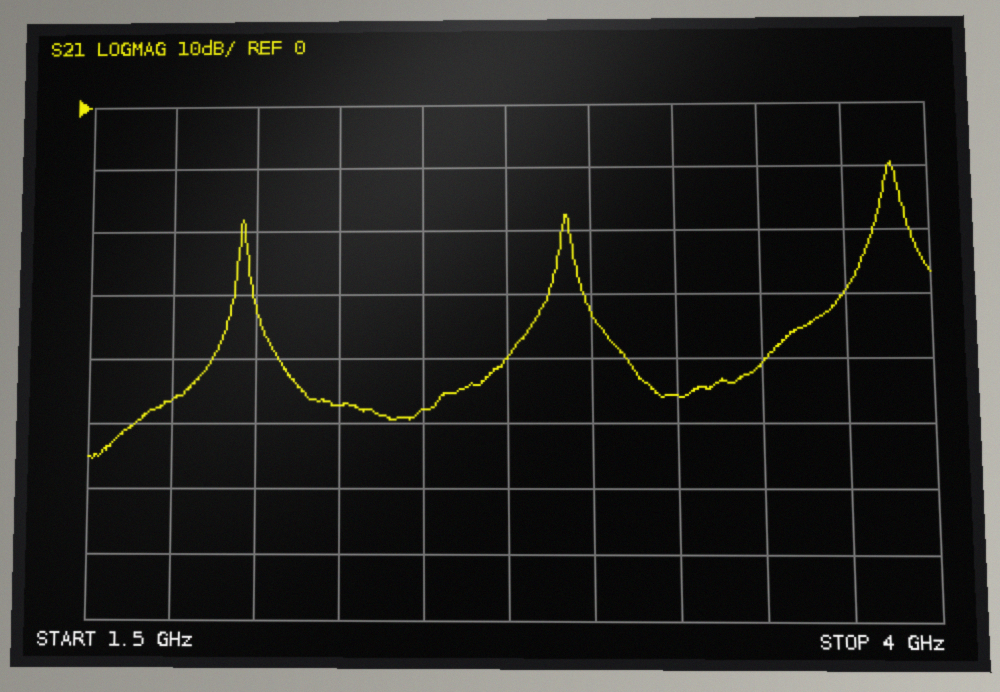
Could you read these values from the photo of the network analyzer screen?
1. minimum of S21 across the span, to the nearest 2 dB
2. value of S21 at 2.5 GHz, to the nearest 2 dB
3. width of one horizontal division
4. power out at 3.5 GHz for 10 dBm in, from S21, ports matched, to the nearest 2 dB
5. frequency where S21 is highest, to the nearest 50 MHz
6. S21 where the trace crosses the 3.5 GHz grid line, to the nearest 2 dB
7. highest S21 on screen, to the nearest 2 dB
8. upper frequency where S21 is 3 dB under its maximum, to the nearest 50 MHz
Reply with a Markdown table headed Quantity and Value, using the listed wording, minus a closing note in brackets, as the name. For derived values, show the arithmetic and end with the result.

| Quantity | Value |
|---|---|
| minimum of S21 across the span, to the nearest 2 dB | -56 dB |
| value of S21 at 2.5 GHz, to the nearest 2 dB | -48 dB |
| width of one horizontal division | 250 MHz |
| power out at 3.5 GHz for 10 dBm in, from S21, ports matched, to the nearest 2 dB | 10 dBm + (-40 dB) = -30 dBm |
| frequency where S21 is highest, to the nearest 50 MHz | 3.90 GHz |
| S21 where the trace crosses the 3.5 GHz grid line, to the nearest 2 dB | -40 dB |
| highest S21 on screen, to the nearest 2 dB | -10 dB |
| upper frequency where S21 is 3 dB under its maximum, to the nearest 50 MHz | 3.90 GHz |
